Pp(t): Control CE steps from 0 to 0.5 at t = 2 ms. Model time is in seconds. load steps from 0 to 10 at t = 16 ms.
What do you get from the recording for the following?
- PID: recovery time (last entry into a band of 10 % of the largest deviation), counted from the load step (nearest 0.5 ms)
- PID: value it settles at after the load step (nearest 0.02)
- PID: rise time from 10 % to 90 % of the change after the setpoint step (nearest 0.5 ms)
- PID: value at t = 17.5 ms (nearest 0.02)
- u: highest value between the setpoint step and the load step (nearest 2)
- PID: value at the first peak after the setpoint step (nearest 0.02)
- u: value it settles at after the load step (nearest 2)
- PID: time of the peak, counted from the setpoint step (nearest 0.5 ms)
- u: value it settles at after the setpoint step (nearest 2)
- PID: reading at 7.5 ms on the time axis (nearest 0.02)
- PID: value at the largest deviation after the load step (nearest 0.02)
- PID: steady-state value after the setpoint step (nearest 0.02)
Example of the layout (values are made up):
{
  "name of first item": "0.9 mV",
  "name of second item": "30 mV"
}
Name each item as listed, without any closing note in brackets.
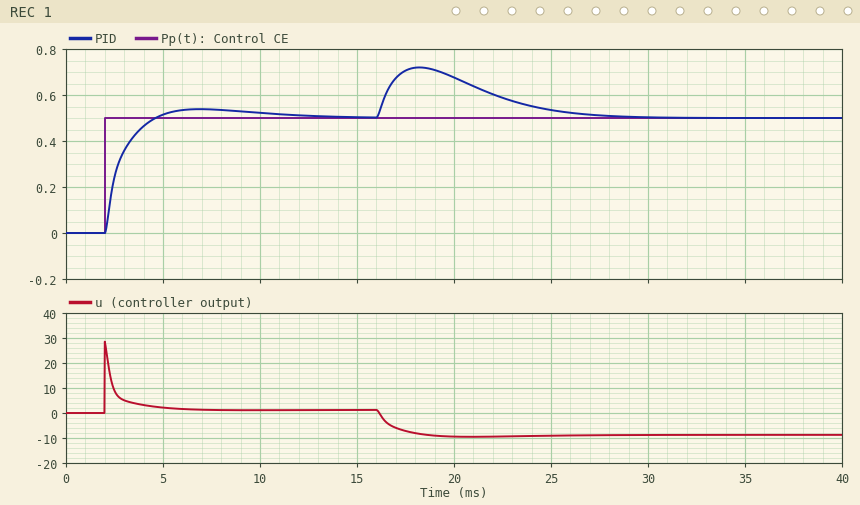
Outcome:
{
  "PID: recovery time (last entry into a band of 10 % of the largest deviation), counted from the load step": "10.0 ms",
  "PID: value it settles at after the load step": "0.50",
  "PID: rise time from 10 % to 90 % of the change after the setpoint step": "1.5 ms",
  "PID: value at t = 17.5 ms": "0.70",
  "u: highest value between the setpoint step and the load step": "28",
  "PID: value at the first peak after the setpoint step": "0.54",
  "u: value it settles at after the load step": "-8",
  "PID: time of the peak, counted from the setpoint step": "5.0 ms",
  "u: value it settles at after the setpoint step": "2",
  "PID: reading at 7.5 ms on the time axis": "0.54",
  "PID: value at the largest deviation after the load step": "0.72",
  "PID: steady-state value after the setpoint step": "0.50"
}
